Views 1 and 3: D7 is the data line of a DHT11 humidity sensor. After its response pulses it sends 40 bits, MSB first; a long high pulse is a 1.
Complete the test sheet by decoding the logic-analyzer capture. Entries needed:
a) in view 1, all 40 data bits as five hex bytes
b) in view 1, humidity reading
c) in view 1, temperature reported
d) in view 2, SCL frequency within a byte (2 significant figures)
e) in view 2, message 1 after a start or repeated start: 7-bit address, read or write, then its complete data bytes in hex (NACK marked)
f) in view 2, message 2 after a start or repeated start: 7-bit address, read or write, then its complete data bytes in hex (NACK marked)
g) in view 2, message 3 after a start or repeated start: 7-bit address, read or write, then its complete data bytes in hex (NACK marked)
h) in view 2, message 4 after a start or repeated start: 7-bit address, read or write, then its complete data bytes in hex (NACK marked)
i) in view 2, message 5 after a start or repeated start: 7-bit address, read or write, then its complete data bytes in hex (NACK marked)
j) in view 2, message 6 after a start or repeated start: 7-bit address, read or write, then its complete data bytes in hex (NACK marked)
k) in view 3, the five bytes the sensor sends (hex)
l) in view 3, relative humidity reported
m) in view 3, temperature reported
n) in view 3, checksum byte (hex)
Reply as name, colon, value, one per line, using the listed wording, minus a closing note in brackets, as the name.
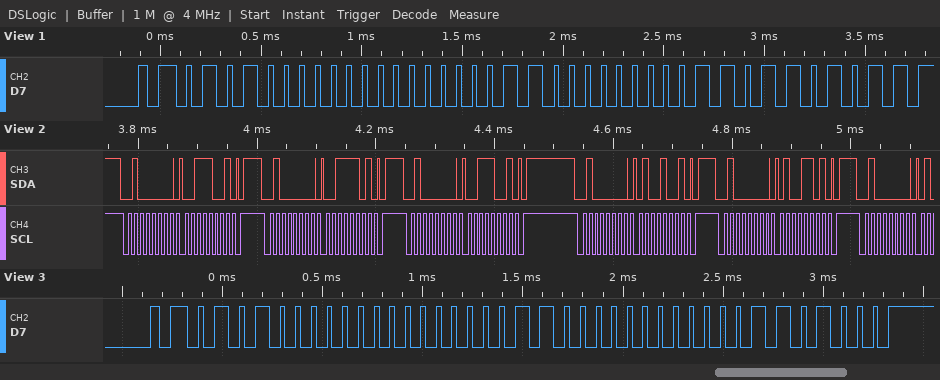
in view 1, all 40 data bits as five hex bytes: 50 00 18 03 6B
in view 1, humidity reading: 80 %
in view 1, temperature reported: 24.3 °C
in view 2, SCL frequency within a byte: 100 kHz
in view 2, message 1 after a start or repeated start: 7-bit address, read or write, then its complete data bytes in hex: 0x20 write: 39
in view 2, message 2 after a start or repeated start: 7-bit address, read or write, then its complete data bytes in hex: 0x20 write: 3D
in view 2, message 3 after a start or repeated start: 7-bit address, read or write, then its complete data bytes in hex: 0x20 write: 39
in view 2, message 4 after a start or repeated start: 7-bit address, read or write, then its complete data bytes in hex: 0x20 write: 49
in view 2, message 5 after a start or repeated start: 7-bit address, read or write, then its complete data bytes in hex: 0x20 write: 4D
in view 2, message 6 after a start or repeated start: 7-bit address, read or write, then its complete data bytes in hex: 0x20 write
in view 3, the five bytes the sensor sends: 50 00 18 00 68
in view 3, relative humidity reported: 80 %
in view 3, temperature reported: 24.0 °C
in view 3, checksum byte: 0x68
